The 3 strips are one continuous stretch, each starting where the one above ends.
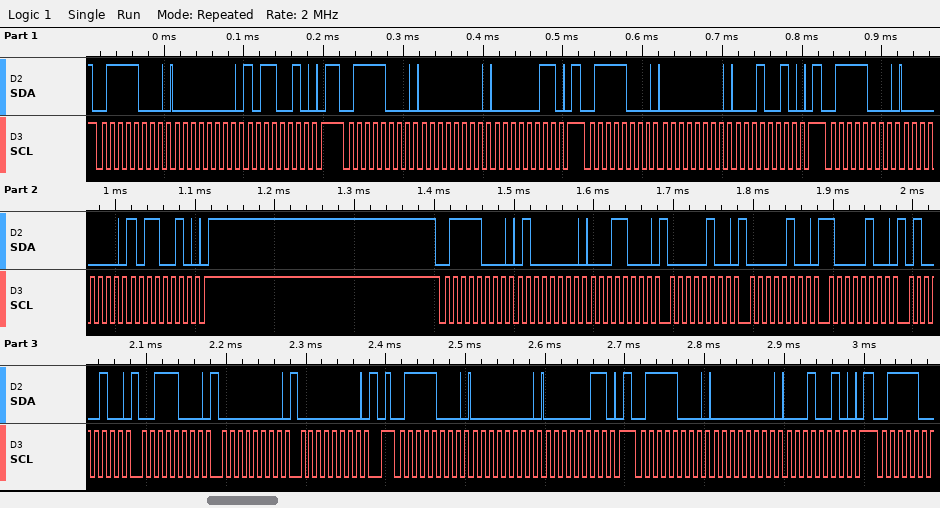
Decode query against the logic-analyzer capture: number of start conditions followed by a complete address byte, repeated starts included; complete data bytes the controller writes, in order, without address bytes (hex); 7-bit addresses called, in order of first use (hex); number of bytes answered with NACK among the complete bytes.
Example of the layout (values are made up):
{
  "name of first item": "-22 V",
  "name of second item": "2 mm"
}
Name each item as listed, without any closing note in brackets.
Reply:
{
  "number of start conditions followed by a complete address byte, repeated starts included": "7",
  "complete data bytes the controller writes, in order, without address bytes": "00 B2 00 03 00 12 00 B2 40 18 04 04 84 44 38 00 00 00 03 00 12",
  "7-bit addresses called, in order of first use": "0x3C",
  "number of bytes answered with NACK among the complete bytes": "0"
}
